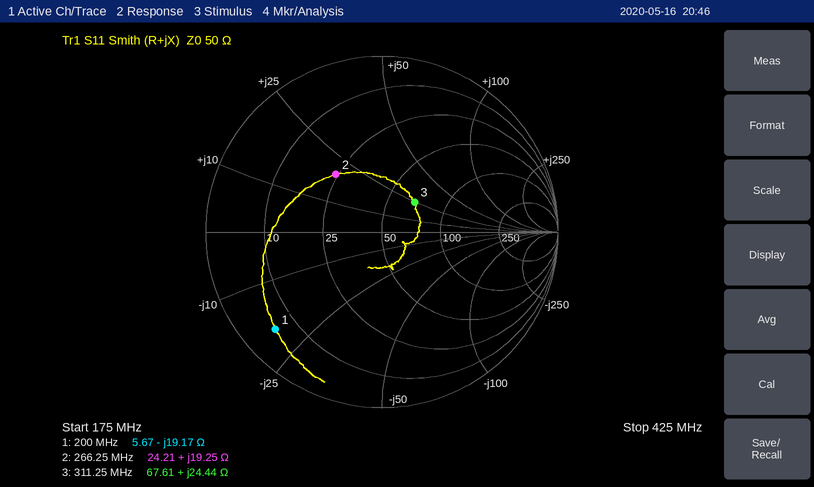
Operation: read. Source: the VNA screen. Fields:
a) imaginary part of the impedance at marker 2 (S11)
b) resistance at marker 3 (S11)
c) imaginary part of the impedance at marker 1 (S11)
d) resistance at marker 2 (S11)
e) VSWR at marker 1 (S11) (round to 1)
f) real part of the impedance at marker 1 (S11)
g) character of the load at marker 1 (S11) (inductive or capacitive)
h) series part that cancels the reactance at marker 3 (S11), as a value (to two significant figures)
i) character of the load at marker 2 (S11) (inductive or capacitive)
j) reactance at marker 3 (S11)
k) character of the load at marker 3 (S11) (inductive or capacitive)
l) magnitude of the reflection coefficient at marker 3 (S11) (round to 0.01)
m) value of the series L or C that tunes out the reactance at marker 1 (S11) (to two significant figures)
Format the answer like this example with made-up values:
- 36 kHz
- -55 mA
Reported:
- +19.25 Ω
- 67.61 Ω
- -19.17 Ω
- 24.21 Ω
- 10
- 5.67 Ω
- capacitive
- 21 pF
- inductive
- +24.44 Ω
- inductive
- 0.25
- 15 nH
